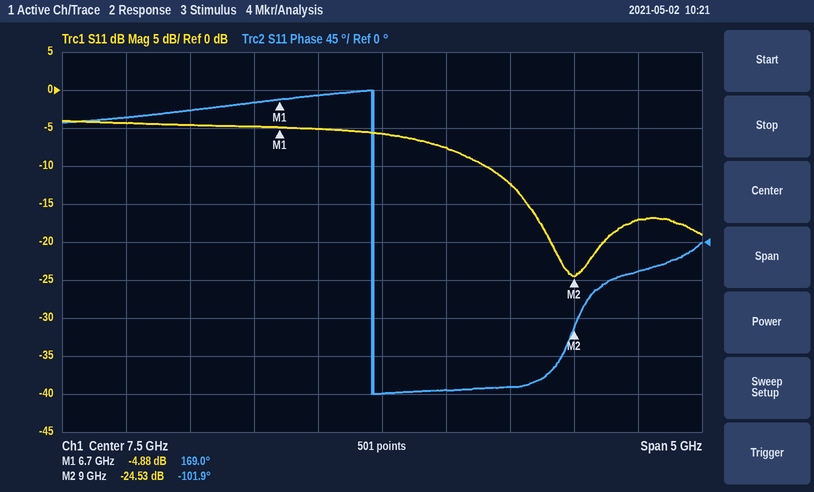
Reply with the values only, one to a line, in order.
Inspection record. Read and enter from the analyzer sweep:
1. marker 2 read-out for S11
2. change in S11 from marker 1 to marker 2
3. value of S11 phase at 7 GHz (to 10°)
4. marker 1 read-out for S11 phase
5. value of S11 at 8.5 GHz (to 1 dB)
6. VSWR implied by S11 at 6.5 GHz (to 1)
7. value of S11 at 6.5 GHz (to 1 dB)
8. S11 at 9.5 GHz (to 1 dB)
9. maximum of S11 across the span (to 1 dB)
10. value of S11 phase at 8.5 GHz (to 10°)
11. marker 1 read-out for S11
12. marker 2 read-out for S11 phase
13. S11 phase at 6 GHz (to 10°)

-24.53 dB
-19.65 dB
170°
169.0°
-12 dB
4
-5 dB
-17 dB
-4 dB
-170°
-4.88 dB
-101.9°
160°
